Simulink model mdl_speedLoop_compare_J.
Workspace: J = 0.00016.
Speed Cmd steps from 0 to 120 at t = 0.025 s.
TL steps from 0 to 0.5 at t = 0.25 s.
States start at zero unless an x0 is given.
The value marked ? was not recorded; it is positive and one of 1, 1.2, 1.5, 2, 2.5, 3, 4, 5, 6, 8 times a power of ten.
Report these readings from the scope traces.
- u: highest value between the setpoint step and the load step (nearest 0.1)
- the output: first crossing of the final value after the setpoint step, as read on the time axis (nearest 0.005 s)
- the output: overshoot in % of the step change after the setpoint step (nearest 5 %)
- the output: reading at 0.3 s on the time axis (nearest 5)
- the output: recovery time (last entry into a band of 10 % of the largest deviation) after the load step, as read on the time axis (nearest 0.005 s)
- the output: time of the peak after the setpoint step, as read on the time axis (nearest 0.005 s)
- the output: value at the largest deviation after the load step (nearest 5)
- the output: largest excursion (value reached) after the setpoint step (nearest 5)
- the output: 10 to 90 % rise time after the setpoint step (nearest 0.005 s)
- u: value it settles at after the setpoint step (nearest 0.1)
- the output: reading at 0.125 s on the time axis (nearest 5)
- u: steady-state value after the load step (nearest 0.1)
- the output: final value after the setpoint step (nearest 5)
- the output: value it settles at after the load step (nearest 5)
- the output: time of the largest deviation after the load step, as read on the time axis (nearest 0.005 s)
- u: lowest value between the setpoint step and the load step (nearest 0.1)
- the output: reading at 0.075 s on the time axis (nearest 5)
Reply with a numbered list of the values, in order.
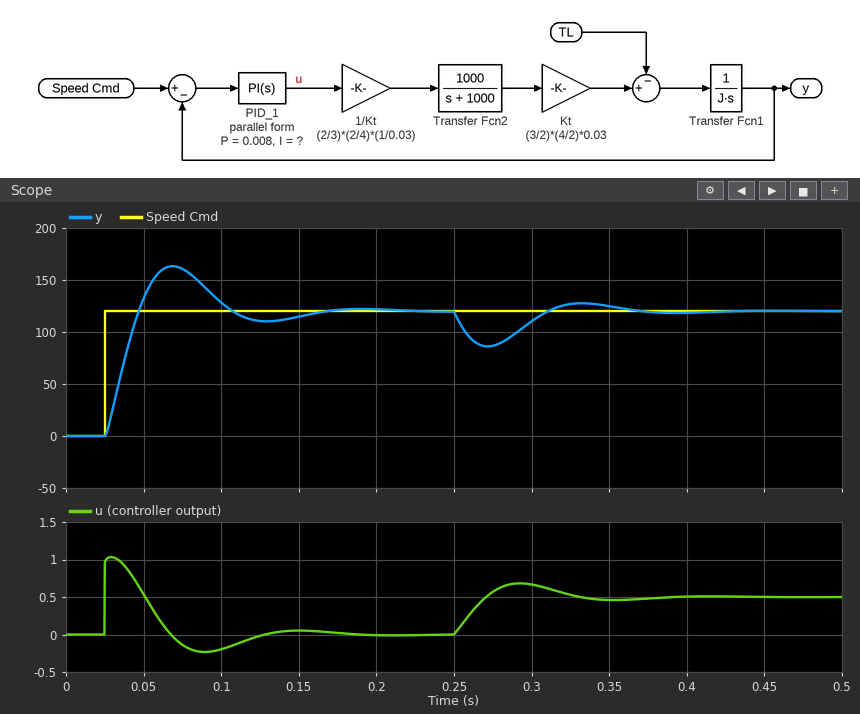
1. 1.0
2. 0.045 s
3. 35 %
4. 110
5. 0.355 s
6. 0.070 s
7. 85
8. 165
9. 0.015 s
10. 0.0
11. 110
12. 0.5
13. 120
14. 120
15. 0.270 s
16. -0.2
17. 160
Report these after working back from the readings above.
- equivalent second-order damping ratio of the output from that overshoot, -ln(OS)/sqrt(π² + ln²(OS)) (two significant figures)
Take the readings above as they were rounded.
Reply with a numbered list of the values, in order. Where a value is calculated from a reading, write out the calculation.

1. ln(0.35) = -1.050; 1.050 / sqrt(9.870 + 1.102) = 0.32
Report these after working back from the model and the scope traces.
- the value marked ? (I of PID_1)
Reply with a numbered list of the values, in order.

1. 0.5
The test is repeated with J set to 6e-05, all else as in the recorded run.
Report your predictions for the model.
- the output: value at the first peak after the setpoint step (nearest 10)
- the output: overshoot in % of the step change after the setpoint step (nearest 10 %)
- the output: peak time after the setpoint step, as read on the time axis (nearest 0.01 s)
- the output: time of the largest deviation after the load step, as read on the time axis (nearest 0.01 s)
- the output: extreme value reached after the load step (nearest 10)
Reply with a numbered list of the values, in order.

1. 150
2. 20 %
3. 0.05 s
4. 0.26 s
5. 80
